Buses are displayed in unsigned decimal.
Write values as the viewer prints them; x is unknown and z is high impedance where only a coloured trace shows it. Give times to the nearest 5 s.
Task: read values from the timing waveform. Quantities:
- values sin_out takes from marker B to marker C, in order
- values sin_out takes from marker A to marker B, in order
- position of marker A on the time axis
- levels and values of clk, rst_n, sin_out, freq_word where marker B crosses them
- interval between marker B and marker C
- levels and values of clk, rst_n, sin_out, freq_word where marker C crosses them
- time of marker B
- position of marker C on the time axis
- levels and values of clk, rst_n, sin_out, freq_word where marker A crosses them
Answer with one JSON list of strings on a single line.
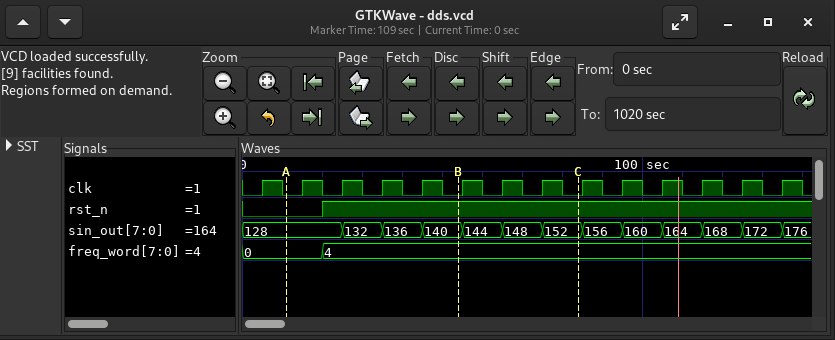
["140, 144, 148, 152", "128, 132, 136, 140", "10 s", "clk=0, rst_n=1, sin_out=140, freq_word=4", "30 s", "clk=0, rst_n=1, sin_out=152, freq_word=4", "55 s", "85 s", "clk=0, rst_n=0, sin_out=128, freq_word=0"]
